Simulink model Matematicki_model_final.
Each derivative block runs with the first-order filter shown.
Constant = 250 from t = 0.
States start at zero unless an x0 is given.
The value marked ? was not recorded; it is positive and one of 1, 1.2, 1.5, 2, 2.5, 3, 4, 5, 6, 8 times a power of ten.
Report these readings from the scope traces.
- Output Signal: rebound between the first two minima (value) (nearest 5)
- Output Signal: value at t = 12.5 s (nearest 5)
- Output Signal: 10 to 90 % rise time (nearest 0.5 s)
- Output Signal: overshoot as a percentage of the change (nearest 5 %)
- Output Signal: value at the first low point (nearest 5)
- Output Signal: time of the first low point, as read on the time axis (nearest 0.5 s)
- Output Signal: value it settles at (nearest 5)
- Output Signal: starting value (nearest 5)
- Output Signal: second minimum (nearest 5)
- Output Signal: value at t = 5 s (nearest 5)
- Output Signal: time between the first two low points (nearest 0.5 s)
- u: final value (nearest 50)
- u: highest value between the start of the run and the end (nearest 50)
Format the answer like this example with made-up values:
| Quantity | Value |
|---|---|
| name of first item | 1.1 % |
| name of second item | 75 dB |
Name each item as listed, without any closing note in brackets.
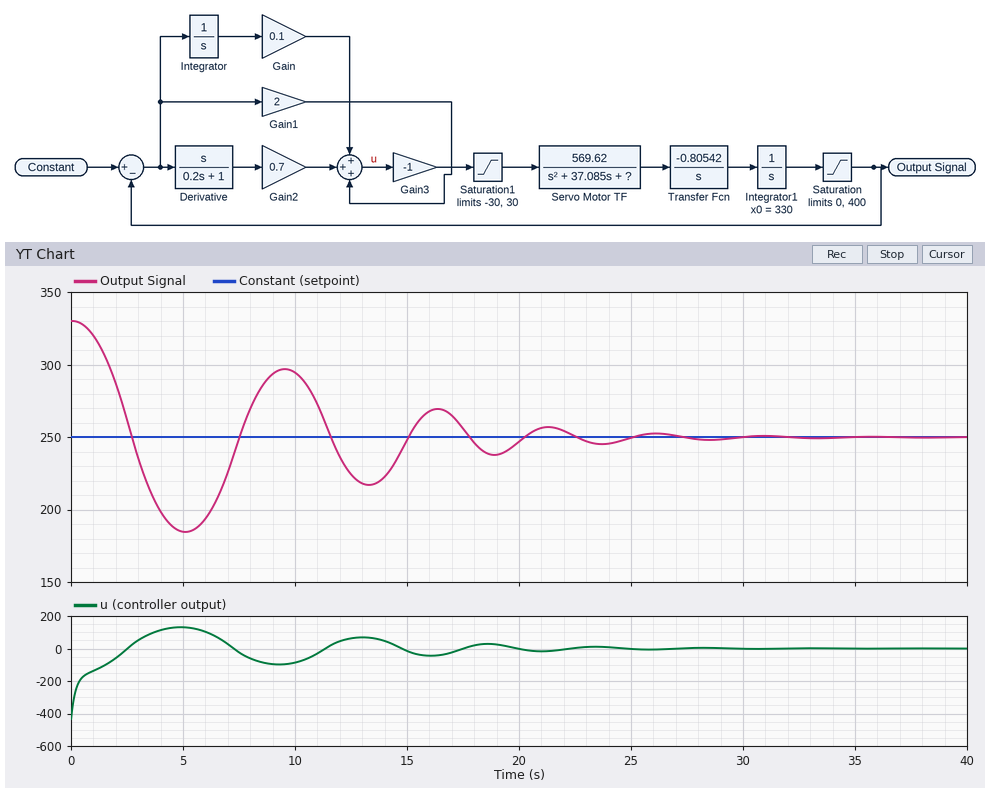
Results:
| Quantity | Value |
|---|---|
| Output Signal: rebound between the first two minima (value) | 295 |
| Output Signal: value at t = 12.5 s | 225 |
| Output Signal: 10 to 90 % rise time | 1.5 s |
| Output Signal: overshoot as a percentage of the change | 80 % |
| Output Signal: value at the first low point | 185 |
| Output Signal: time of the first low point, as read on the time axis | 5.0 s |
| Output Signal: value it settles at | 250 |
| Output Signal: starting value | 330 |
| Output Signal: second minimum | 215 |
| Output Signal: value at t = 5 s | 185 |
| Output Signal: time between the first two low points | 8.0 s |
| u: final value | 0 |
| u: highest value between the start of the run and the end | 150 |
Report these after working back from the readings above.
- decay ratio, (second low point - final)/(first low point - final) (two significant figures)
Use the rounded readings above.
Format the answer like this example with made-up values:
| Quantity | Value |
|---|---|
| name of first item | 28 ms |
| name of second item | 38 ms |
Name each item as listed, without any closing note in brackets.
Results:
| Quantity | Value |
|---|---|
| decay ratio, (second low point - final)/(first low point - final) | 0.54 |
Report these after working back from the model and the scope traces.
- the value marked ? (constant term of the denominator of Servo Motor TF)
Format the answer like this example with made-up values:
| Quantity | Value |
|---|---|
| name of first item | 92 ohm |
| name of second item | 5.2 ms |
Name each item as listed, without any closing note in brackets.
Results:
| Quantity | Value |
|---|---|
| the value marked ? | 600 |
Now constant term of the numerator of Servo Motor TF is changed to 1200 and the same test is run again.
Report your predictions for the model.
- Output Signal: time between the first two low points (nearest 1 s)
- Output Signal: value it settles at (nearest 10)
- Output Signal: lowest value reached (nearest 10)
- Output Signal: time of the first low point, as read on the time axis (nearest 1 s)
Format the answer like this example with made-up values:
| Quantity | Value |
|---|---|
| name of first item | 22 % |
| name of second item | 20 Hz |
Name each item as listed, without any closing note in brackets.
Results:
| Quantity | Value |
|---|---|
| Output Signal: time between the first two low points | 4 s |
| Output Signal: value it settles at | 250 |
| Output Signal: lowest value reached | 200 |
| Output Signal: time of the first low point, as read on the time axis | 3 s |
